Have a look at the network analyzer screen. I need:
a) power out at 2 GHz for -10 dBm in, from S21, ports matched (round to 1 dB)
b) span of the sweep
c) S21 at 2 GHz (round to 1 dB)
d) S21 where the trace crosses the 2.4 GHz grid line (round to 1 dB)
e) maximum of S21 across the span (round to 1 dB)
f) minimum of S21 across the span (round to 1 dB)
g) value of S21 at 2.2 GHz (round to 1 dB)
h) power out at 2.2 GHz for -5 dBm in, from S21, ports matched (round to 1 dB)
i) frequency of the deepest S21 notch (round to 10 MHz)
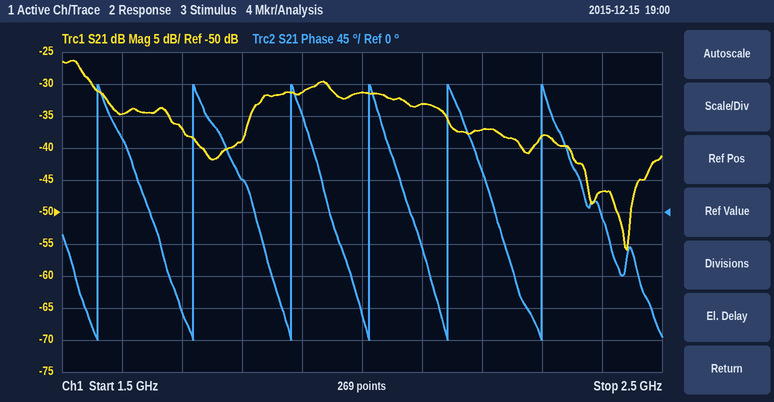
-41 dBm
1 GHz
-31 dB
-47 dB
-26 dB
-56 dB
-37 dB
-42 dBm
2.44 GHz
